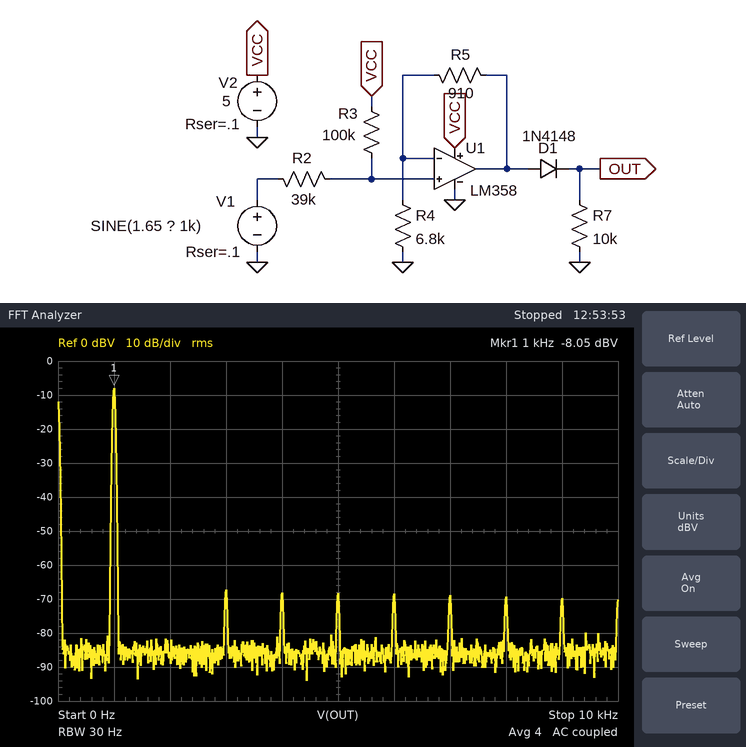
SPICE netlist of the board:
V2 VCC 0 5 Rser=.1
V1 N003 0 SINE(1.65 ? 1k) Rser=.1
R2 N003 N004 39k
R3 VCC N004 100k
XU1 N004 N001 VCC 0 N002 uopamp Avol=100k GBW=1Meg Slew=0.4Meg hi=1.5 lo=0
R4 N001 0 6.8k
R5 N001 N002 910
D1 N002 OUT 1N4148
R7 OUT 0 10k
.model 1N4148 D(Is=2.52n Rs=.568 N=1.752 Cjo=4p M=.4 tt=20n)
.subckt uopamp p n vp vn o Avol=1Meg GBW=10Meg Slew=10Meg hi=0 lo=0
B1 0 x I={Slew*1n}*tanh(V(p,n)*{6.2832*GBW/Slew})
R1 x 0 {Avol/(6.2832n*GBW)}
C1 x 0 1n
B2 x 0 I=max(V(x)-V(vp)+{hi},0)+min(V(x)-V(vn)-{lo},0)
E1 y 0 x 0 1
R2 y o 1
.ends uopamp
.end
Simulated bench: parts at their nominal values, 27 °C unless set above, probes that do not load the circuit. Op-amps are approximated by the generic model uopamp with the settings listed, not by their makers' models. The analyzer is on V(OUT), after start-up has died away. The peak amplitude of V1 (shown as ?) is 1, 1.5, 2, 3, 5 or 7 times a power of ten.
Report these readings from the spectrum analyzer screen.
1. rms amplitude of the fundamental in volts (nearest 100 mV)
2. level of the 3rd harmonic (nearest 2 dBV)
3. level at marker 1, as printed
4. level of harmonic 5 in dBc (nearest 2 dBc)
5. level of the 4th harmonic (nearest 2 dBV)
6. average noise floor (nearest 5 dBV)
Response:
400 mV
-68 dBV
-8.05 dBV
-60 dBc
-68 dBV
-85 dBV
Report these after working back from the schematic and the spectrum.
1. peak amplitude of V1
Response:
700 mV
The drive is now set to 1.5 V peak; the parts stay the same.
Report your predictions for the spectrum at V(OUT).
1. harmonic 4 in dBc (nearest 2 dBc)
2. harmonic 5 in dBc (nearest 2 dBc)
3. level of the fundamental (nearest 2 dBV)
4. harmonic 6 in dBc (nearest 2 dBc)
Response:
-40 dBc
-32 dBc
-4 dBV
-34 dBc
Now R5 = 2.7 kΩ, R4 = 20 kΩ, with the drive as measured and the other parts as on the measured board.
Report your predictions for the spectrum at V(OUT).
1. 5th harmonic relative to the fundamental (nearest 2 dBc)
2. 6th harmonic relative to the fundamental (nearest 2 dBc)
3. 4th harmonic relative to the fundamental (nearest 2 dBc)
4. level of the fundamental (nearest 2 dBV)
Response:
-56 dBc
-56 dBc
-56 dBc
-8 dBV
